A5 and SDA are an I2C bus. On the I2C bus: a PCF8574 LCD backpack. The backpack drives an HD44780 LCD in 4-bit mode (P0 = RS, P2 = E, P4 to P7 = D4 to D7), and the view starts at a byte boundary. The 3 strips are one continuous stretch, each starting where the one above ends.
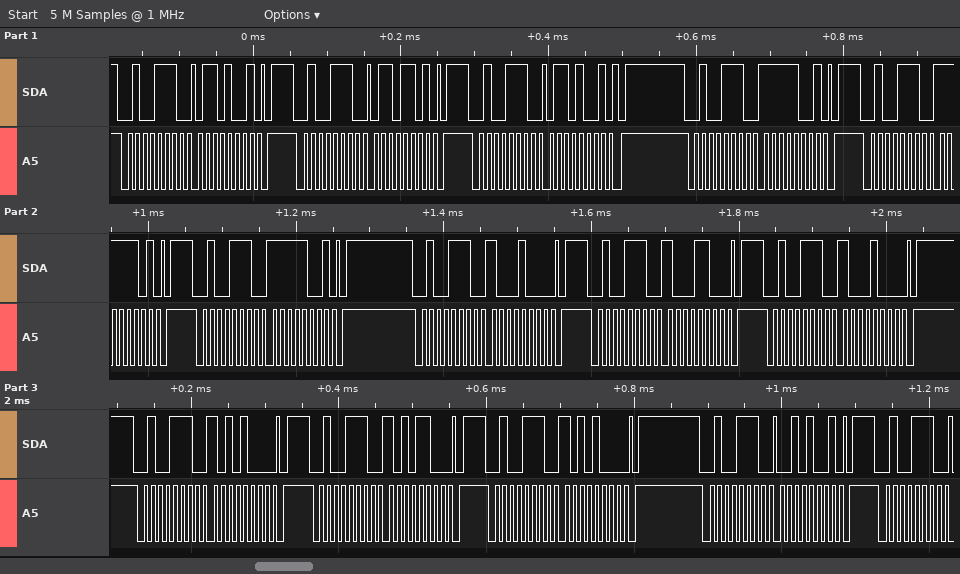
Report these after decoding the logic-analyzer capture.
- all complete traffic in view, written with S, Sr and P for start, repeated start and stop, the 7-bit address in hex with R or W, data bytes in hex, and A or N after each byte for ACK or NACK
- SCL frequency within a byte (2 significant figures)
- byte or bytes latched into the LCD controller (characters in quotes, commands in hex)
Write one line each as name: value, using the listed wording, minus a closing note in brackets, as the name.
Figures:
all complete traffic in view, written with S, Sr and P for start, repeated start and stop, the 7-bit address in hex with R or W, data bytes in hex, and A or N after each byte for ACK or NACK: S 27W A 69 A P S 27W A 6D A P S 27W A 69 A P S 27W A F9 A P S 27W A FD A P S 27W A F9 A P S 27W A 88 A P S 27W A 8C A P S 27W A 88 A P S 27W A A8 A P S 27W A AC A P S 27W A A8 A P S 27W A 29 A P S 27W A
SCL frequency within a byte: 100 kHz
byte or bytes latched into the LCD controller: 'o' 0x8A
